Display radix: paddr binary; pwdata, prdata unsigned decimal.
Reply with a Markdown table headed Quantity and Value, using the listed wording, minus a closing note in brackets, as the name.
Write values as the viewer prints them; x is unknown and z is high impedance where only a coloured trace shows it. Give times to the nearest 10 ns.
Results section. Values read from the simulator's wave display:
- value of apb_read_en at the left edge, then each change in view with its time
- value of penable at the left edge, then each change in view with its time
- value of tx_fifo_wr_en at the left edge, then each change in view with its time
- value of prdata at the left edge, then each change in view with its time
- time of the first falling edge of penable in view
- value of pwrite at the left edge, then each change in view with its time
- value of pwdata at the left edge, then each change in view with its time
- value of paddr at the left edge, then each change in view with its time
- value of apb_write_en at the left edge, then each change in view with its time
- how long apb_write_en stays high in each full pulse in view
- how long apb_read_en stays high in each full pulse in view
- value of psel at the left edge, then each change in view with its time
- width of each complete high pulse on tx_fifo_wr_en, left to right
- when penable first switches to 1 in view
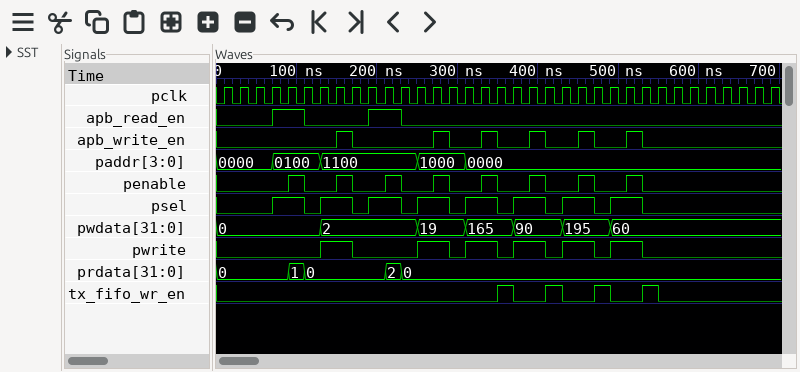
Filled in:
| Quantity | Value |
|---|---|
| value of apb_read_en at the left edge, then each change in view with its time | 0, 1 at 70 ns, 0 at 110 ns, 1 at 190 ns, 0 at 230 ns |
| value of penable at the left edge, then each change in view with its time | 0, 1 at 90 ns, 0 at 110 ns, 1 at 150 ns, 0 at 170 ns, 1 at 210 ns, 0 at 230 ns, 1 at 270 ns, 0 at 290 ns, 1 at 330 ns, 0 at 350 ns, 1 at 390 ns, 0 at 410 ns, 1 at 450 ns, 0 at 470 ns, 1 at 510 ns, 0 at 530 ns |
| value of tx_fifo_wr_en at the left edge, then each change in view with its time | 0, 1 at 350 ns, 0 at 370 ns, 1 at 410 ns, 0 at 430 ns, 1 at 470 ns, 0 at 490 ns, 1 at 530 ns, 0 at 550 ns |
| value of prdata at the left edge, then each change in view with its time | 0, 1 at 90 ns, 0 at 110 ns, 2 at 210 ns, 0 at 230 ns |
| time of the first falling edge of penable in view | 110 ns |
| value of pwrite at the left edge, then each change in view with its time | 0, 1 at 130 ns, 0 at 170 ns, 1 at 250 ns, 0 at 290 ns, 1 at 310 ns, 0 at 350 ns, 1 at 370 ns, 0 at 410 ns, 1 at 430 ns, 0 at 470 ns, 1 at 490 ns, 0 at 530 ns |
| value of pwdata at the left edge, then each change in view with its time | 0, 2 at 130 ns, 19 at 250 ns, 165 at 310 ns, 90 at 370 ns, 195 at 430 ns, 60 at 490 ns |
| value of paddr at the left edge, then each change in view with its time | 0000, 0100 at 70 ns, 1100 at 130 ns, 1000 at 250 ns, 0000 at 310 ns |
| value of apb_write_en at the left edge, then each change in view with its time | 0, 1 at 150 ns, 0 at 170 ns, 1 at 270 ns, 0 at 290 ns, 1 at 330 ns, 0 at 350 ns, 1 at 390 ns, 0 at 410 ns, 1 at 450 ns, 0 at 470 ns, 1 at 510 ns, 0 at 530 ns |
| how long apb_write_en stays high in each full pulse in view | 20 ns, 20 ns, 20 ns, 20 ns, 20 ns, 20 ns |
| how long apb_read_en stays high in each full pulse in view | 40 ns, 40 ns |
| value of psel at the left edge, then each change in view with its time | 0, 1 at 70 ns, 0 at 110 ns, 1 at 130 ns, 0 at 170 ns, 1 at 190 ns, 0 at 230 ns, 1 at 250 ns, 0 at 290 ns, 1 at 310 ns, 0 at 350 ns, 1 at 370 ns, 0 at 410 ns, 1 at 430 ns, 0 at 470 ns, 1 at 490 ns, 0 at 530 ns |
| width of each complete high pulse on tx_fifo_wr_en, left to right | 20 ns, 20 ns, 20 ns, 20 ns |
| when penable first switches to 1 in view | 90 ns |
